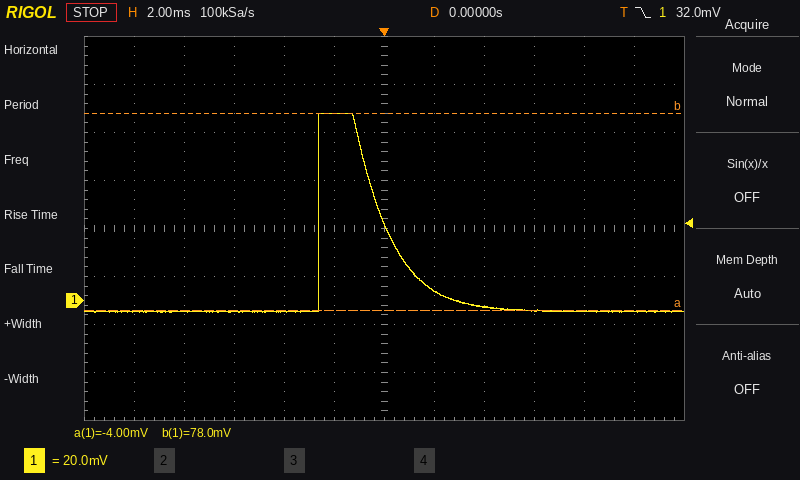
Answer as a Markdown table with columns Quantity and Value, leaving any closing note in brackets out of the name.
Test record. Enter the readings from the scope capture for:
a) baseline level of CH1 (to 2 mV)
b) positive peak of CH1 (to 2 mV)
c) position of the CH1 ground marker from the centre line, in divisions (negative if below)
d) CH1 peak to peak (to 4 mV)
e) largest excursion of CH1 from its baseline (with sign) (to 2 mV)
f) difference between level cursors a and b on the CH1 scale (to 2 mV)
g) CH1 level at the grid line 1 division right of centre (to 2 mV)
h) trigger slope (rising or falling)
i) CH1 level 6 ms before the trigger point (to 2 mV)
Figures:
| Quantity | Value |
|---|---|
| baseline level of CH1 | -4 mV |
| positive peak of CH1 | 78 mV |
| position of the CH1 ground marker from the centre line, in divisions | -1.5 div |
| CH1 peak to peak | 84 mV |
| largest excursion of CH1 from its baseline (with sign) | +82 mV |
| difference between level cursors a and b on the CH1 scale | 82 mV |
| CH1 level at the grid line 1 division right of centre | 4 mV |
| trigger slope | falling |
| CH1 level 6 ms before the trigger point | -4 mV |
